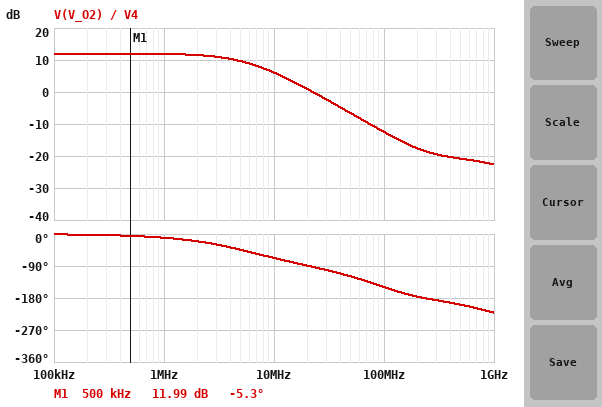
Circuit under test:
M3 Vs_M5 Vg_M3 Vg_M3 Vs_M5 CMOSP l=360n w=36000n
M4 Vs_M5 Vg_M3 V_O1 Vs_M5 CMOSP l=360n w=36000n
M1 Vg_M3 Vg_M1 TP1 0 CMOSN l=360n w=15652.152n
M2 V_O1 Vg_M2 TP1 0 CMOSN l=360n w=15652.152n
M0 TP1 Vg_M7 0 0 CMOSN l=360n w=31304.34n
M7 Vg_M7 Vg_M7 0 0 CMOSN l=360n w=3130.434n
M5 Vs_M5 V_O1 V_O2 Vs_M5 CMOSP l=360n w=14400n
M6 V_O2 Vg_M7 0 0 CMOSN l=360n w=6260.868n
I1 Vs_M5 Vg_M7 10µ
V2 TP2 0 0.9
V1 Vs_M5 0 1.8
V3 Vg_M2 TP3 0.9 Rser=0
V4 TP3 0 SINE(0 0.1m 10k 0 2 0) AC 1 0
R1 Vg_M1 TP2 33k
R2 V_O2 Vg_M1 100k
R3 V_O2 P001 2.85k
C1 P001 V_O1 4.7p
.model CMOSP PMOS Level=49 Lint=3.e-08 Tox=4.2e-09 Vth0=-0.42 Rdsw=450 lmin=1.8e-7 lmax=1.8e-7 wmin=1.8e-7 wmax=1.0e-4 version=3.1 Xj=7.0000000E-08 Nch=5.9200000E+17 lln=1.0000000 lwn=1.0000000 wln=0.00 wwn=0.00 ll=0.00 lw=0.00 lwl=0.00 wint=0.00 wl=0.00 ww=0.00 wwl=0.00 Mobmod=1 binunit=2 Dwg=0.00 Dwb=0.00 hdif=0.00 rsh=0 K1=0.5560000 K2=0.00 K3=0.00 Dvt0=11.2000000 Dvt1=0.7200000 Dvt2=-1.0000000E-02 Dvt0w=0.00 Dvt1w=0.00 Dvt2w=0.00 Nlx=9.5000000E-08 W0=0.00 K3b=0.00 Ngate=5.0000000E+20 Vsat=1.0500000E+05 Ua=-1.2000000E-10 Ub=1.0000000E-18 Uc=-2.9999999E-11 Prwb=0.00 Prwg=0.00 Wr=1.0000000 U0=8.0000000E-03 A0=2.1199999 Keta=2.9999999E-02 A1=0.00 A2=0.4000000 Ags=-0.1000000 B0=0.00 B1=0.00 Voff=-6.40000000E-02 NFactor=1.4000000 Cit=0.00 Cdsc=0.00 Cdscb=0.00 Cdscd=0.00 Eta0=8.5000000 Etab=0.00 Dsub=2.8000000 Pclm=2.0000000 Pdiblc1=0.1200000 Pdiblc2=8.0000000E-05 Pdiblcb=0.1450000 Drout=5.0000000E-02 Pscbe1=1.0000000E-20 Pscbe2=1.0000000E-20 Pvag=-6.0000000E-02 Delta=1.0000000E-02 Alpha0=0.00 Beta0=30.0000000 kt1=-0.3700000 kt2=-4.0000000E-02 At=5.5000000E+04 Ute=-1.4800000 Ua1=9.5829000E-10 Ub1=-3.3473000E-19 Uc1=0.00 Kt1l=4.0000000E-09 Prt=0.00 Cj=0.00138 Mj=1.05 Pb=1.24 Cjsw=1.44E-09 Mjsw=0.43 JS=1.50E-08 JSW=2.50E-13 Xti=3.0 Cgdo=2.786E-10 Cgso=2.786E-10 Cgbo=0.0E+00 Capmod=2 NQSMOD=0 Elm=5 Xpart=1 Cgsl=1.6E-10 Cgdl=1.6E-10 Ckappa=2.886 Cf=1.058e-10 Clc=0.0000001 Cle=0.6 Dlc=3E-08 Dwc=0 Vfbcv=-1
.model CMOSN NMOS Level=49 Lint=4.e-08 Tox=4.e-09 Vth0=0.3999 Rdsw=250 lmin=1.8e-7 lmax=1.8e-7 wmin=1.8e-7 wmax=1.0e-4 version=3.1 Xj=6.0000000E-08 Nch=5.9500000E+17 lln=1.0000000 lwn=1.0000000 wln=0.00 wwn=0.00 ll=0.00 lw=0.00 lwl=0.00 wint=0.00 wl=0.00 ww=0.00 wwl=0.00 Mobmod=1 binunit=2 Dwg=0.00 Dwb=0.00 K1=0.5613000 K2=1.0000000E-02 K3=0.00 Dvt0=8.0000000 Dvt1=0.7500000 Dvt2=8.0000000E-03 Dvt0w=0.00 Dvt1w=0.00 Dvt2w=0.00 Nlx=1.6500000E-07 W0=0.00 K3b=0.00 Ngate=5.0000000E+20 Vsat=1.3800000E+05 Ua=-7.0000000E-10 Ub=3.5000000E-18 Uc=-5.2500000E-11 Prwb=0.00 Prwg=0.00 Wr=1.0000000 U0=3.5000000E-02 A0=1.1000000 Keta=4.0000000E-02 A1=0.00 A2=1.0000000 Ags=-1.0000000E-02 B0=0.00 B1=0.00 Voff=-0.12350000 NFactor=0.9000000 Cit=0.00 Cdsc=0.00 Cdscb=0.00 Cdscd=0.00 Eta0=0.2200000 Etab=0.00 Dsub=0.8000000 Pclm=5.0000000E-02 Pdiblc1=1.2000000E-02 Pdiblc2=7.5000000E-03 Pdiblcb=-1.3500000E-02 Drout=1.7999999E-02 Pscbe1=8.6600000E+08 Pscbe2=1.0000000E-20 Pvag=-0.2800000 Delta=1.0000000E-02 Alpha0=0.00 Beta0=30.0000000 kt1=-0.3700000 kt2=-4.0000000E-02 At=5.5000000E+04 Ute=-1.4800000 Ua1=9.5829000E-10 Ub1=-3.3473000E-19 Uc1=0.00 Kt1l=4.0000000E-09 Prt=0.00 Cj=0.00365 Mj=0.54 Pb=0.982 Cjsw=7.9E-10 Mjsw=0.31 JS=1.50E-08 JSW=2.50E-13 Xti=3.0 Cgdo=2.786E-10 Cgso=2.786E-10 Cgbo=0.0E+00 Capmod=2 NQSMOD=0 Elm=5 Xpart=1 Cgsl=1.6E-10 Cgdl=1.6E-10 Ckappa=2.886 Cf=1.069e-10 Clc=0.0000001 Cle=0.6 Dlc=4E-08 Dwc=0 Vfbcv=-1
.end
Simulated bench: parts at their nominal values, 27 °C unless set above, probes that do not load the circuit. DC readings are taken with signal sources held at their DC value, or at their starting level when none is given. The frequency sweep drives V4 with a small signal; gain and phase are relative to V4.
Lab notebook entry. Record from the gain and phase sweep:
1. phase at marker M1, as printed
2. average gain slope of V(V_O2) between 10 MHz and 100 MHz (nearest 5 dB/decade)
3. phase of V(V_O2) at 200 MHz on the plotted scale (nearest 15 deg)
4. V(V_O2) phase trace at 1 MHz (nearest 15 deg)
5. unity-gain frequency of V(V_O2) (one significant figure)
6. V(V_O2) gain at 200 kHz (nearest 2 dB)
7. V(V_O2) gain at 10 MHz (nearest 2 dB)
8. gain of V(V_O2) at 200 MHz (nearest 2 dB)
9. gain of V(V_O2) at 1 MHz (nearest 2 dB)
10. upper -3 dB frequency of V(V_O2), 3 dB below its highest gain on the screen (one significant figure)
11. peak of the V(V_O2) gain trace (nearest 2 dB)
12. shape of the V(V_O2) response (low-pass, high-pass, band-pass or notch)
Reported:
-5.3 deg
-20 dB/decade
-180 deg
-15 deg
20 MHz
12 dB
6 dB
-18 dB
12 dB
6 MHz
12 dB
low-pass
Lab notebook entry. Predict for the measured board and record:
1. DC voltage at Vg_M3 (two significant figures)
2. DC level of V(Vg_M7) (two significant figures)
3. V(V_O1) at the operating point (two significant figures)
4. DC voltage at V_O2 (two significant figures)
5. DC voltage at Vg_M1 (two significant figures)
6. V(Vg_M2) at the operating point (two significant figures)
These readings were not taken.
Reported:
1.2 V
570 mV
1.2 V
900 mV
900 mV
900 mV
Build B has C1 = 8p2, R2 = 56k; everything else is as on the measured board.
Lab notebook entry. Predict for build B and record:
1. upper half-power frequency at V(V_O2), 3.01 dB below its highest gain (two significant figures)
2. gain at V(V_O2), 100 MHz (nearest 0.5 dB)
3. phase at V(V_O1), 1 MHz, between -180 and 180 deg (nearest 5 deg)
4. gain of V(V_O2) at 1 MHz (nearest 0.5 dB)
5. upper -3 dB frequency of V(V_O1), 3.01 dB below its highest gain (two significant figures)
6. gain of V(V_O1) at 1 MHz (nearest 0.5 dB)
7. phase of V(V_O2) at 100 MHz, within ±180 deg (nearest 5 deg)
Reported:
4.9 MHz
-15.5 dB
-125 deg
8.5 dB
150 MHz
-6.5 dB
-160 deg
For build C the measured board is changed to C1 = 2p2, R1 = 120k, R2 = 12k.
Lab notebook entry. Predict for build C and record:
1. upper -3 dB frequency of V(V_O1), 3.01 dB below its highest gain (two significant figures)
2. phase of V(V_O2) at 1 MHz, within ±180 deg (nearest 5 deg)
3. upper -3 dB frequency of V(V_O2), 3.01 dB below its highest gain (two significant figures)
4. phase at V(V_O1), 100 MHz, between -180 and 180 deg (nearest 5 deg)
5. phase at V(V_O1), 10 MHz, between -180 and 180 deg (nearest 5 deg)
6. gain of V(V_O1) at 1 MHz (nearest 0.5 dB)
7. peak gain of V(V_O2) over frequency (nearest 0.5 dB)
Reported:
170 MHz
0 deg
77 MHz
165 deg
-110 deg
-21.5 dB
1.0 dB
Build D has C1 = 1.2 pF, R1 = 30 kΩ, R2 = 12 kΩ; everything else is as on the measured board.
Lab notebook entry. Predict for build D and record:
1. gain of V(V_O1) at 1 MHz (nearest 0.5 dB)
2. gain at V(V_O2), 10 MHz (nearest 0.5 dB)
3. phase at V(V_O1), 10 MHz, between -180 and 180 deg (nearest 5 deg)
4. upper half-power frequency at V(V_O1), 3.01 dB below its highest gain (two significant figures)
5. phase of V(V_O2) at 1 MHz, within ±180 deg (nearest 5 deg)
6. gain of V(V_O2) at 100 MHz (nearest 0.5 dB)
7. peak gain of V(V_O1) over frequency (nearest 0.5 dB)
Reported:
-16.0 dB
3.0 dB
-120 deg
190 MHz
0 deg
0.5 dB
8.5 dB
